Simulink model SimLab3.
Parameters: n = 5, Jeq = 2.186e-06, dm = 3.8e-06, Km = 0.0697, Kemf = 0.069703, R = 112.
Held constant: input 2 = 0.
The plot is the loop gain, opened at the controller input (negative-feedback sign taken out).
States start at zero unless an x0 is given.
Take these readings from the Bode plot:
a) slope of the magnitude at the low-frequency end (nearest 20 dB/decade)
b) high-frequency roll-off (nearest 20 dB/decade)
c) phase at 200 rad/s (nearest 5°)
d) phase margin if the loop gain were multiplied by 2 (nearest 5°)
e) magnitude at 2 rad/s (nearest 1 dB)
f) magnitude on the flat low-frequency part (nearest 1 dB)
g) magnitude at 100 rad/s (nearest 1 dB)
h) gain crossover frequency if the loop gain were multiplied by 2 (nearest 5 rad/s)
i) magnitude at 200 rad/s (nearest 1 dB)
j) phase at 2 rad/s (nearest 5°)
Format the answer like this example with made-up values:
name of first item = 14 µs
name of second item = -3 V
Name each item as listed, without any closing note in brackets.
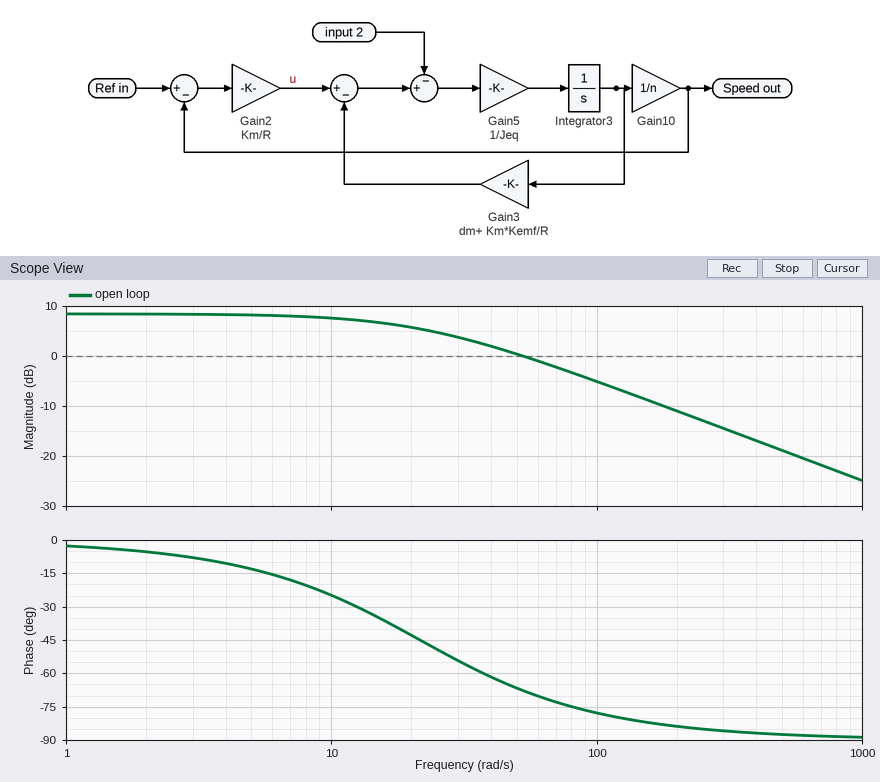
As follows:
slope of the magnitude at the low-frequency end = 0 dB/decade
high-frequency roll-off = -20 dB/decade
phase at 200 rad/s = -85°
phase margin if the loop gain were multiplied by 2 = 100°
magnitude at 2 rad/s = 8 dB
magnitude on the flat low-frequency part = 8 dB
magnitude at 100 rad/s = -5 dB
gain crossover frequency if the loop gain were multiplied by 2 = 110 rad/s
magnitude at 200 rad/s = -11 dB
phase at 2 rad/s = -5°
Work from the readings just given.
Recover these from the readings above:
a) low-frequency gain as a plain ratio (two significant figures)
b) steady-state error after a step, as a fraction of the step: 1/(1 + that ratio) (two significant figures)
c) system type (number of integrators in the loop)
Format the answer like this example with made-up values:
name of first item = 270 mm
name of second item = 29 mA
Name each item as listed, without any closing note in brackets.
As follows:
low-frequency gain as a plain ratio = 2.5
steady-state error after a step, as a fraction of the step: 1/(1 + that ratio) = 0.29
system type = 0
